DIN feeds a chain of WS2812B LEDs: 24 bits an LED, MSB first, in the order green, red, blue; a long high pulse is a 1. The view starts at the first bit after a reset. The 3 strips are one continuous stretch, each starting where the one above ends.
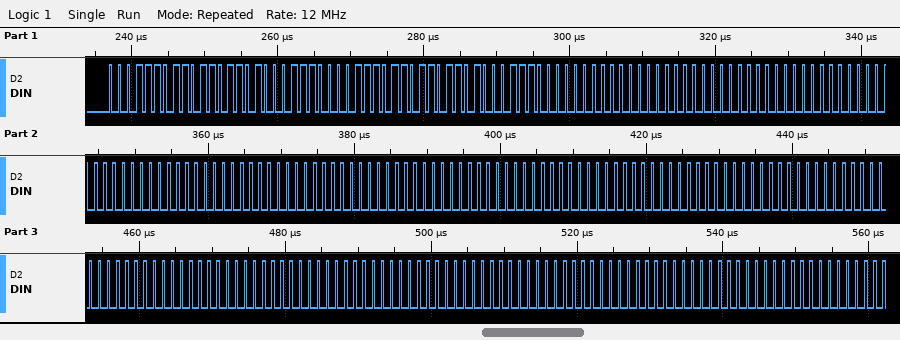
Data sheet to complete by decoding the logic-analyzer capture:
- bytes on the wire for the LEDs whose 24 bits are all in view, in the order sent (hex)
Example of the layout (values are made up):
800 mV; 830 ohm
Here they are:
1D B6 8E 1D B6 8E 00 00 00 00 00 00 00 00 00 00 00 00 00 00 00 00 00 00 00 00 00 00 00 00
